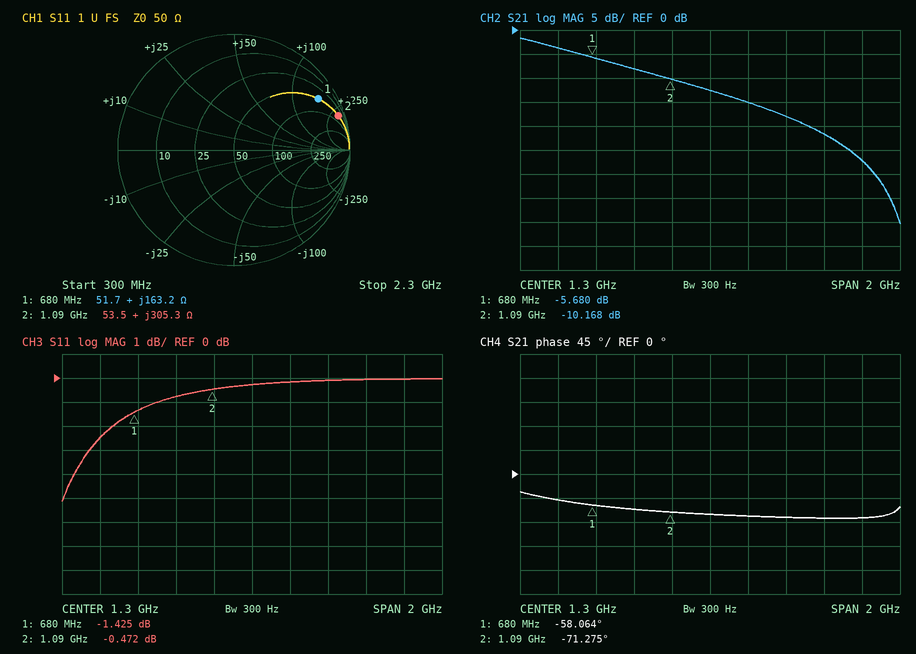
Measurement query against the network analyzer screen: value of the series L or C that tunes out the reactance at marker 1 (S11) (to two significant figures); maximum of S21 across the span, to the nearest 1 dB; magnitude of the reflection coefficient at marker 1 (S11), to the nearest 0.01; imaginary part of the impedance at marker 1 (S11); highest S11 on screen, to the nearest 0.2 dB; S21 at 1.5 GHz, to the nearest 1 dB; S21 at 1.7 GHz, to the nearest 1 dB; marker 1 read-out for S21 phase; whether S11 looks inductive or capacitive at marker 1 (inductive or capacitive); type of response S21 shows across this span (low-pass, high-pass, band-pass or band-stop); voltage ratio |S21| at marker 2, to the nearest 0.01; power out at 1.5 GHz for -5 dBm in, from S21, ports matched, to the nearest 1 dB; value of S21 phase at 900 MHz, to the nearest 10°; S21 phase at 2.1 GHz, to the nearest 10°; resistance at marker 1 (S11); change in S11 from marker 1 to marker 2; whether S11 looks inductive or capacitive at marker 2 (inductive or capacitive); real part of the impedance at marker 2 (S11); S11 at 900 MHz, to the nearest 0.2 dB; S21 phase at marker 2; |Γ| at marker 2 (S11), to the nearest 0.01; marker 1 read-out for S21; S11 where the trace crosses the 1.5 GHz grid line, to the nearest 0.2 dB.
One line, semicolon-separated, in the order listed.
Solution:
1.4 pF; -2 dB; 0.85; +163.2 Ω; 0.0 dB; -15 dB; -18 dB; -58.064°; inductive; low-pass; 0.31; -20 dBm; -70°; -80°; 51.7 Ω; 0.953 dB; inductive; 53.5 Ω; -0.8 dB; -71.275°; 0.95; -5.680 dB; -0.2 dB
